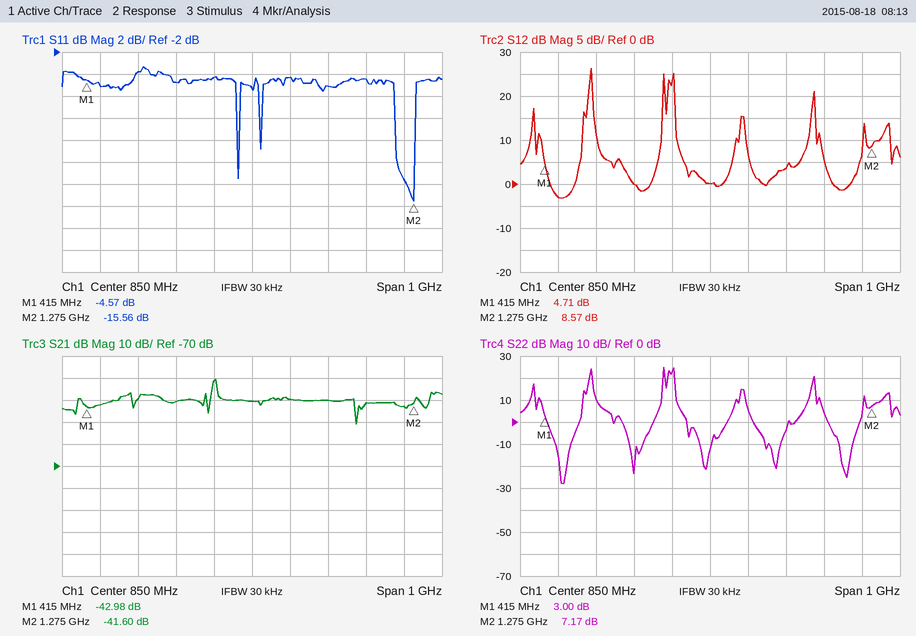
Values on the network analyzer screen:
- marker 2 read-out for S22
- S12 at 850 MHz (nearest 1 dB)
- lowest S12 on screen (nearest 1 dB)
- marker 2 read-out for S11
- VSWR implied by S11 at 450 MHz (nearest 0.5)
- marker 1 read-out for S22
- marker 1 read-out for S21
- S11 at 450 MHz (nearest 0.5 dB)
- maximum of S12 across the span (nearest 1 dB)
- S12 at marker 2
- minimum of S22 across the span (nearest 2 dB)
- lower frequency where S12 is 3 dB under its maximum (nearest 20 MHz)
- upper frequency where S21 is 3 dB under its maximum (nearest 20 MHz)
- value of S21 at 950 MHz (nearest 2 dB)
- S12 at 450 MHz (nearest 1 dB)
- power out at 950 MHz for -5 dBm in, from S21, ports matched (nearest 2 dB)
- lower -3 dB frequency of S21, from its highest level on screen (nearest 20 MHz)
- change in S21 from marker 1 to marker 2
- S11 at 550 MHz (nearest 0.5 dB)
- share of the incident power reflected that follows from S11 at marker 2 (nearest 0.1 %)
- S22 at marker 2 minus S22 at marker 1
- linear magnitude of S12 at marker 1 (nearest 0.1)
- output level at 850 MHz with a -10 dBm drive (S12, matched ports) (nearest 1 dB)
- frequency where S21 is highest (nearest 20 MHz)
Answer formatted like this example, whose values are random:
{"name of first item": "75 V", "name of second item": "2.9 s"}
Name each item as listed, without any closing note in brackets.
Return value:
{"marker 2 read-out for S22": "7.17 dB", "S12 at 850 MHz": "0 dB", "lowest S12 on screen": "-3 dB", "marker 2 read-out for S11": "-15.56 dB", "VSWR implied by S11 at 450 MHz": "3.5", "marker 1 read-out for S22": "3.00 dB", "marker 1 read-out for S21": "-42.98 dB", "S11 at 450 MHz": "-5.0 dB", "maximum of S12 across the span": "26 dB", "S12 at marker 2": "8.57 dB", "minimum of S22 across the span": "-28 dB", "lower frequency where S12 is 3 dB under its maximum": "540 MHz", "upper frequency where S21 is 3 dB under its maximum": "760 MHz", "value of S21 at 950 MHz": "-40 dB", "S12 at 450 MHz": "-3 dB", "power out at 950 MHz for -5 dBm in, from S21, ports matched": "-44 dBm", "lower -3 dB frequency of S21, from its highest level on screen": "740 MHz", "change in S21 from marker 1 to marker 2": "1.38 dB", "S11 at 550 MHz": "-4.0 dB", "share of the incident power reflected that follows from S11 at marker 2": "2.8 %", "S22 at marker 2 minus S22 at marker 1": "4.17 dB", "linear magnitude of S12 at marker 1": "1.7", "output level at 850 MHz with a -10 dBm drive (S12, matched ports)": "-10 dBm", "frequency where S21 is highest": "760 MHz"}
